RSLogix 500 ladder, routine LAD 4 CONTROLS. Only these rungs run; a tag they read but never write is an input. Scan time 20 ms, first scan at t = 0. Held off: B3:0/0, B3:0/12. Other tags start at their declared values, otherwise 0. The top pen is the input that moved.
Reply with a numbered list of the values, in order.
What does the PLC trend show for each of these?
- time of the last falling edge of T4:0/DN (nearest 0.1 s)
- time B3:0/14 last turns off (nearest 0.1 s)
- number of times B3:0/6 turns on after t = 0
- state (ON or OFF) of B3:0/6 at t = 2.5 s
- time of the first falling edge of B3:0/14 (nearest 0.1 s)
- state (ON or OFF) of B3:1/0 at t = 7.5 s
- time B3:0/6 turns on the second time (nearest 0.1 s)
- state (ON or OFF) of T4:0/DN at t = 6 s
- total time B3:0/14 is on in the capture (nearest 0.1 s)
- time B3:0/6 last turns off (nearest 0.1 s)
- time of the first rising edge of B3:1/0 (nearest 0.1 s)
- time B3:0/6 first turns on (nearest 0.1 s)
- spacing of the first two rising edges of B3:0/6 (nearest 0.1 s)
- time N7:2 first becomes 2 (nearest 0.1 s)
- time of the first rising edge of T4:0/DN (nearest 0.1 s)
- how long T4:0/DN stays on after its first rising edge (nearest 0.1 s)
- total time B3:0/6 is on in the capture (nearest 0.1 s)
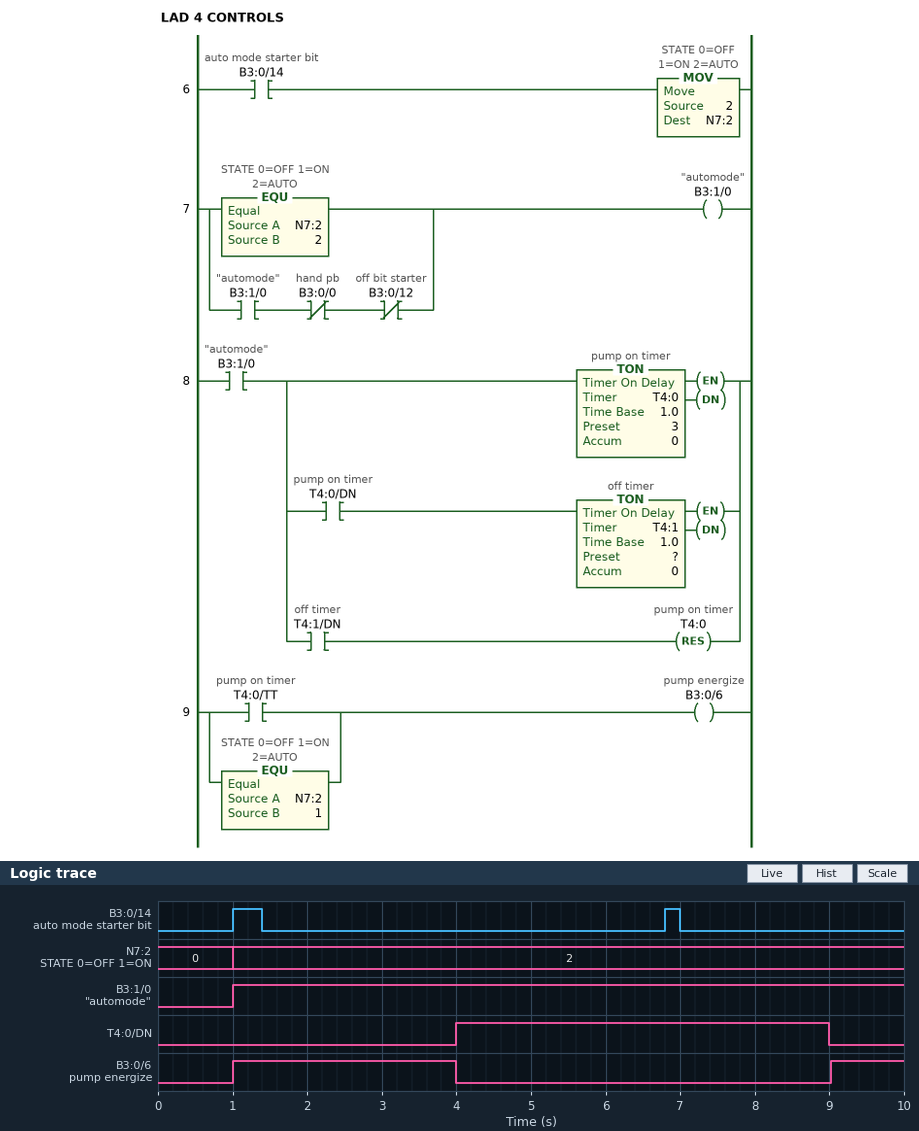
1. 9.0 s
2. 7.0 s
3. 2
4. ON
5. 1.4 s
6. ON
7. 9.0 s
8. ON
9. 0.6 s
10. 4.0 s
11. 1.0 s
12. 1.0 s
13. 8.0 s
14. 1.0 s
15. 4.0 s
16. 5.0 s
17. 4.0 s
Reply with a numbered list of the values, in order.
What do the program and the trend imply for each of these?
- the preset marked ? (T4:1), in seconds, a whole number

1. 5 s
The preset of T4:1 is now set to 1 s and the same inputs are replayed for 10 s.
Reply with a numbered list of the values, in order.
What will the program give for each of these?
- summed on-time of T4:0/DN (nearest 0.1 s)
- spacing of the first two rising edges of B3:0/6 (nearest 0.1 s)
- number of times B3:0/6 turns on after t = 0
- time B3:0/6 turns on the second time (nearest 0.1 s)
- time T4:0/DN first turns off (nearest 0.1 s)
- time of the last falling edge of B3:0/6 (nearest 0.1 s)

1. 2.0 s
2. 4.0 s
3. 3
4. 5.0 s
5. 5.0 s
6. 8.0 s
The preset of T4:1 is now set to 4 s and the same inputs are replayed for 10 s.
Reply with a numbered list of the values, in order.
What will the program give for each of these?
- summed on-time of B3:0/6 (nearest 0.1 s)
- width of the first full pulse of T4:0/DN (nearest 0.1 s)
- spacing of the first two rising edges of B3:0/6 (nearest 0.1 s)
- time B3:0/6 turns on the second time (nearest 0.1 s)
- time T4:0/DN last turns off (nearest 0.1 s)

1. 5.0 s
2. 4.0 s
3. 7.0 s
4. 8.0 s
5. 8.0 s
